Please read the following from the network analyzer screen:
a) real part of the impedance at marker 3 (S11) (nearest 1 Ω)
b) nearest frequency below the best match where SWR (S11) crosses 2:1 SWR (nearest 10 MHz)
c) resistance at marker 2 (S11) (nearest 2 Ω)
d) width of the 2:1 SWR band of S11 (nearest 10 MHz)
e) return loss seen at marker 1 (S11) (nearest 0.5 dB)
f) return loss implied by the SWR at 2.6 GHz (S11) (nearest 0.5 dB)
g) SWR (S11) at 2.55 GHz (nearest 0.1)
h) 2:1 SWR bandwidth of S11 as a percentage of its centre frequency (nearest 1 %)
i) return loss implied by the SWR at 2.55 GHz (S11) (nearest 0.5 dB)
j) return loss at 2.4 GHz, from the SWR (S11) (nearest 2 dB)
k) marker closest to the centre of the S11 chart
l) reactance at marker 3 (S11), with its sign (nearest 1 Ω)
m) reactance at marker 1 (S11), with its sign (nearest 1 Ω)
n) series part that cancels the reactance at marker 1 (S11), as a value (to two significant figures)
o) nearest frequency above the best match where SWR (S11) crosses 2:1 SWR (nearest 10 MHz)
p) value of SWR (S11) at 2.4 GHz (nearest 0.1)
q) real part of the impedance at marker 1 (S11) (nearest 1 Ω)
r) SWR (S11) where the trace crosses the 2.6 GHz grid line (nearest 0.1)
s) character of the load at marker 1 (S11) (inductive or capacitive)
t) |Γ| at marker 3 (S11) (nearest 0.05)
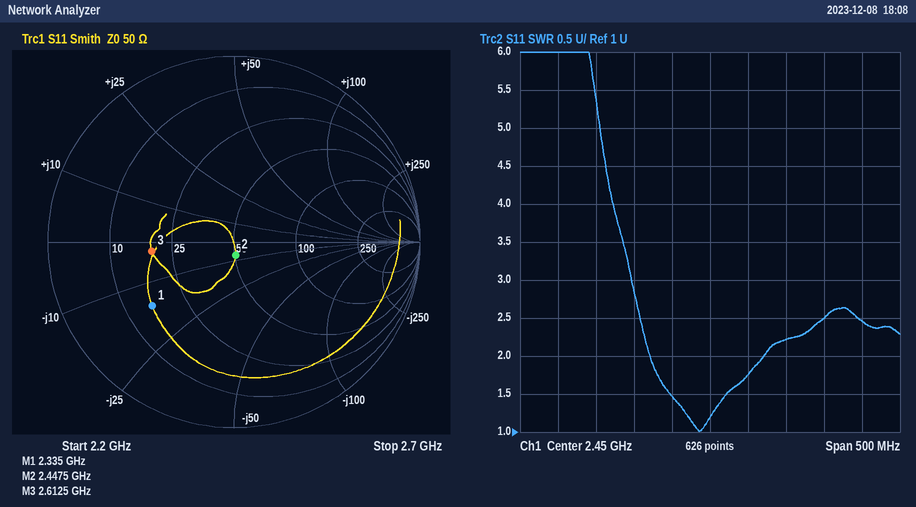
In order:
19 Ω
2.37 GHz
50 Ω
150 MHz
5.0 dB
7.5 dB
2.2
6 %
8.5 dB
14 dB
marker 2
-2 Ω
-16 Ω
1.1 nH
2.52 GHz
1.5
16 Ω
2.5
capacitive
0.45
